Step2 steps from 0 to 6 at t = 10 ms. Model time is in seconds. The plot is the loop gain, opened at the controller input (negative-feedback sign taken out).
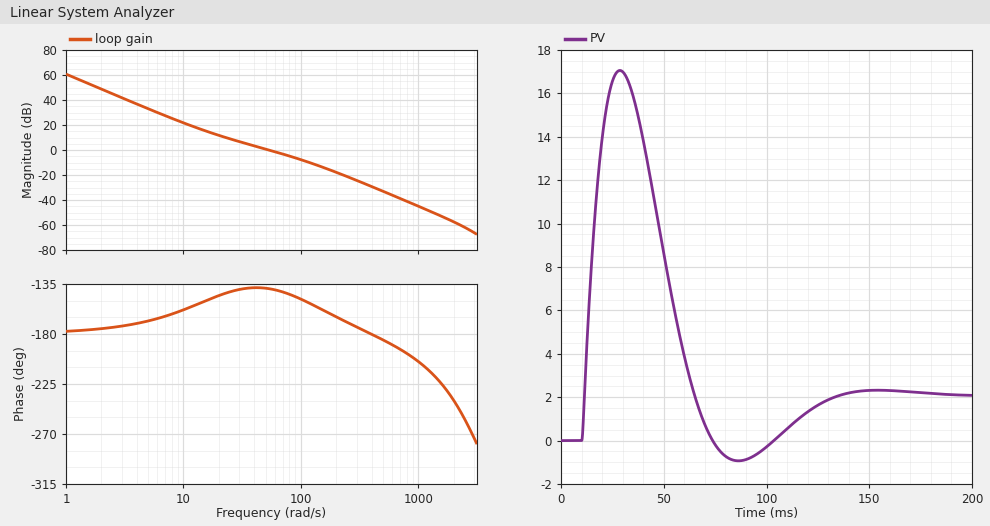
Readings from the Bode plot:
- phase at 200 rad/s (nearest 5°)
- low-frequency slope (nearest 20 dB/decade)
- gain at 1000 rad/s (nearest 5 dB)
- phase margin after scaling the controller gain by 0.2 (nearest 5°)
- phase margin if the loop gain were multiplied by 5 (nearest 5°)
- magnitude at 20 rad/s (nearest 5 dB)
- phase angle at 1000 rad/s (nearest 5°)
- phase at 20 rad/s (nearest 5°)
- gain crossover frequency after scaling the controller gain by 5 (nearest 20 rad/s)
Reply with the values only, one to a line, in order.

-165°
-40 dB/decade
-45 dB
30°
20°
10 dB
-205°
-145°
160 rad/s
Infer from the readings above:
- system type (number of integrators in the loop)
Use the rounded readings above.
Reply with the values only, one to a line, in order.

2
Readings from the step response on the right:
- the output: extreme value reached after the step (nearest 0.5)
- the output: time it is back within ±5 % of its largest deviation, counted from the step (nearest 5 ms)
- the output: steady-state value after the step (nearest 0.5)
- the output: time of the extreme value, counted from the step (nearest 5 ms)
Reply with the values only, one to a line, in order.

17.0
110 ms
2.0
20 ms
